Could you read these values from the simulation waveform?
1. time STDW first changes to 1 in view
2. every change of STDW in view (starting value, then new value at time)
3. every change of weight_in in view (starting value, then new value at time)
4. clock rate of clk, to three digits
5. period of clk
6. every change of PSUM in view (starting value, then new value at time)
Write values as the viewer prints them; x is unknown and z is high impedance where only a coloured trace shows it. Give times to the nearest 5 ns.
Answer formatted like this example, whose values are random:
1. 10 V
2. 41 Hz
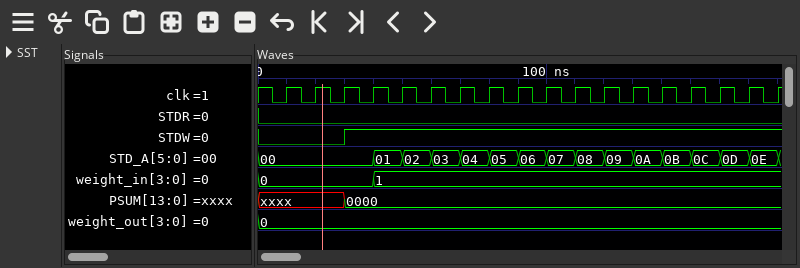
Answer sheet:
1. 30 ns
2. 0, 1 at 30 ns
3. 0, 1 at 40 ns
4. 100 MHz
5. 10 ns
6. xxxx, 0000 at 30 ns
